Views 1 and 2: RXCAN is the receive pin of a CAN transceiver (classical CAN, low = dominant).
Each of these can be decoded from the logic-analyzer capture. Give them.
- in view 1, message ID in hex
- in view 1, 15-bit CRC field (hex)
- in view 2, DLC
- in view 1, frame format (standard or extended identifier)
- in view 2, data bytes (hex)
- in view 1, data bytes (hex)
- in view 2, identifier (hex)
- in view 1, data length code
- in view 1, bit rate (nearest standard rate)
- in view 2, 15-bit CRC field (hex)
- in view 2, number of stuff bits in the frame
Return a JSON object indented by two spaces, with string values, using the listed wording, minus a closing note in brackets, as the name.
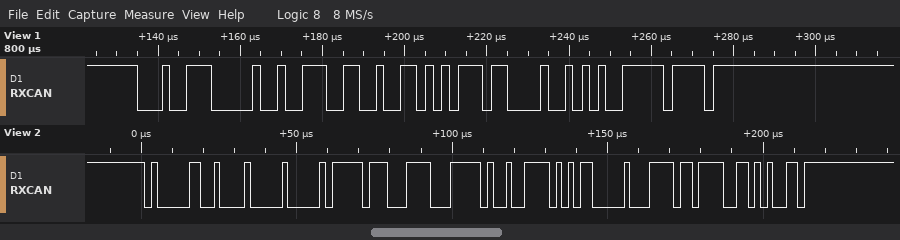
{
  "in view 1, message ID in hex": "0x138",
  "in view 1, 15-bit CRC field": "0x54FF",
  "in view 2, DLC": "8",
  "in view 1, frame format": "standard",
  "in view 2, data bytes": "00 FF 1E 3F 27 AB 00 F6",
  "in view 1, data bytes": "E6 4D 5D 84",
  "in view 2, identifier": "0x412",
  "in view 1, data length code": "4",
  "in view 1, bit rate": "500 kbit/s",
  "in view 2, 15-bit CRC field": "0x79A9",
  "in view 2, number of stuff bits in the frame": "6"
}
